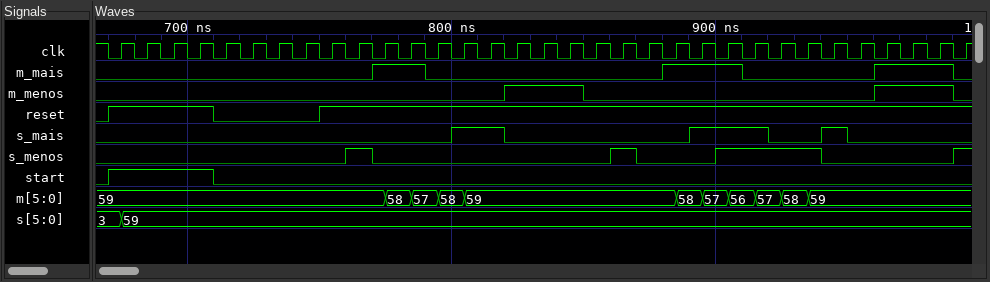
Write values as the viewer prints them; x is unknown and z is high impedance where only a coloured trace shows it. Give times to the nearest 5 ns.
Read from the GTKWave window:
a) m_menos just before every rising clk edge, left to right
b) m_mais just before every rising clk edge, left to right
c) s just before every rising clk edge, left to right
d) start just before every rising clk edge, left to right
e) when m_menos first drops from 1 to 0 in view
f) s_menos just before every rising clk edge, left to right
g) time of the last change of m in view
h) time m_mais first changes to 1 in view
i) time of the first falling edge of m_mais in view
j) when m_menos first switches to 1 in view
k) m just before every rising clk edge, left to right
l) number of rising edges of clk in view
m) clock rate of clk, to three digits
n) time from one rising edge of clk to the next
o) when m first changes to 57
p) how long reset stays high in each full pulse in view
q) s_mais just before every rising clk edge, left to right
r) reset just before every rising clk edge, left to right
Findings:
0 0 0 0 0 0 0 0 0 0 0 0 0 0 0 1 1 1 0 0 0 0 0 0 0 0 0 0 0 1 1 1 0
0 0 0 0 0 0 0 0 0 0 1 1 0 0 0 0 0 0 0 0 0 1 1 1 0 0 0 0 0 1 1 1 0
3, 59, 59, 59, 59, 59, 59, 59, 59, 59, 59, 59, 59, 59, 59, 59, 59, 59, 59, 59, 59, 59, 59, 59, 59, 59, 59, 59, 59, 59, 59, 59, 59
1 1 1 1 0 0 0 0 0 0 0 0 0 0 0 0 0 0 0 0 0 0 0 0 0 0 0 0 0 0 0 0 0
850 ns
0 0 0 0 0 0 0 0 0 1 0 0 0 0 0 0 0 0 0 1 0 0 0 1 1 1 1 0 0 0 0 0 1
935 ns
770 ns
790 ns
820 ns
59, 59, 59, 59, 59, 59, 59, 59, 59, 59, 59, 58, 57, 58, 59, 59, 59, 59, 59, 59, 59, 59, 58, 57, 56, 57, 58, 59, 59, 59, 59, 59, 59
33
100 MHz
10 ns
785 ns
40 ns
0 0 0 0 0 0 0 0 0 0 0 0 0 1 1 0 0 0 0 0 0 0 1 1 1 0 0 1 0 0 0 0 0
1 1 1 1 0 0 0 0 1 1 1 1 1 1 1 1 1 1 1 1 1 1 1 1 1 1 1 1 1 1 1 1 1
